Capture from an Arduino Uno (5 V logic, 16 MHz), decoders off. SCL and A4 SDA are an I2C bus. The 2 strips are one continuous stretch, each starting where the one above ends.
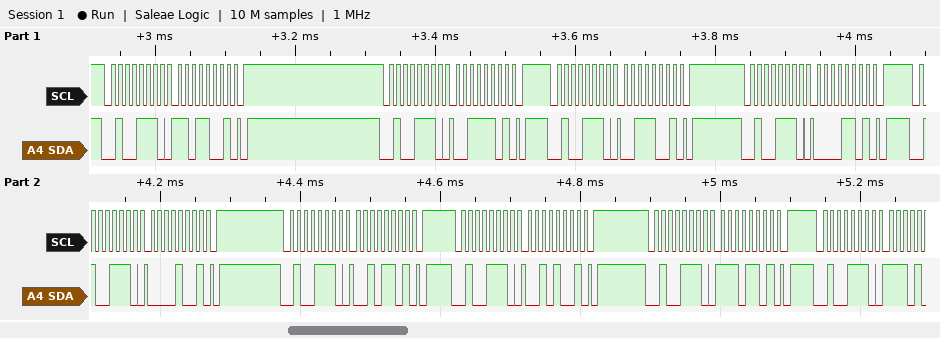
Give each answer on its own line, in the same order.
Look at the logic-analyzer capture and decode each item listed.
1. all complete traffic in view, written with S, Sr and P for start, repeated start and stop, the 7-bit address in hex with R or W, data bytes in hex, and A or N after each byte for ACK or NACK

S 27W A D9 A P S 27W A 3D A P S 27W A 39 A P S 27W A 0D A P S 27W A 09 A P S 27W A 2D A P S 27W A 29 A P S 27W A ED A P S 27W A
